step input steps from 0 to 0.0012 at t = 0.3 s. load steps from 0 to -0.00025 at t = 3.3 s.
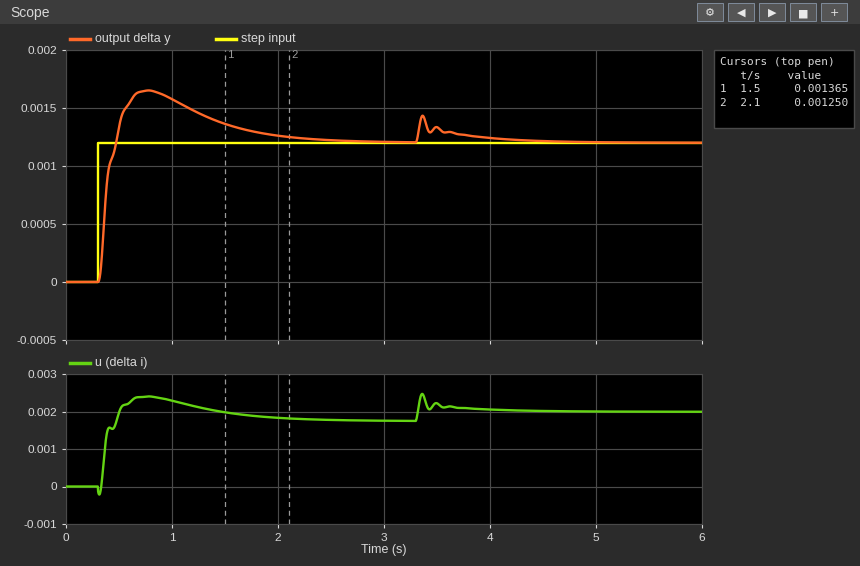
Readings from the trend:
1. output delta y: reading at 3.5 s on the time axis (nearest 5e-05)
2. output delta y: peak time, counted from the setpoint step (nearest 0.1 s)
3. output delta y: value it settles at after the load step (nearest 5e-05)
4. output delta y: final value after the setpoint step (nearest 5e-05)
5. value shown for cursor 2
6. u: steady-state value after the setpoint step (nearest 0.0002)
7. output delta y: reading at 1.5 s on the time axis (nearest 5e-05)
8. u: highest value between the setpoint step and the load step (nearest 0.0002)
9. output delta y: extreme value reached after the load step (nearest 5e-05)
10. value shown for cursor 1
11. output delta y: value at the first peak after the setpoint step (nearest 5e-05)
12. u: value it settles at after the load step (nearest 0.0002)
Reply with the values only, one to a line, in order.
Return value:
0.00135
0.5 s
0.00120
0.00120
0.001250
0.0018
0.00135
0.0024
0.00145
0.001365
0.00165
0.0020
